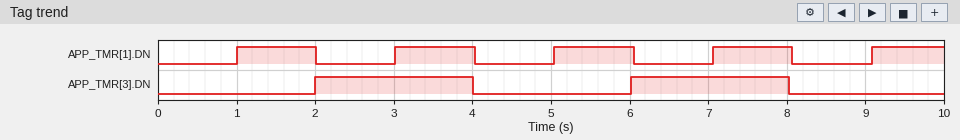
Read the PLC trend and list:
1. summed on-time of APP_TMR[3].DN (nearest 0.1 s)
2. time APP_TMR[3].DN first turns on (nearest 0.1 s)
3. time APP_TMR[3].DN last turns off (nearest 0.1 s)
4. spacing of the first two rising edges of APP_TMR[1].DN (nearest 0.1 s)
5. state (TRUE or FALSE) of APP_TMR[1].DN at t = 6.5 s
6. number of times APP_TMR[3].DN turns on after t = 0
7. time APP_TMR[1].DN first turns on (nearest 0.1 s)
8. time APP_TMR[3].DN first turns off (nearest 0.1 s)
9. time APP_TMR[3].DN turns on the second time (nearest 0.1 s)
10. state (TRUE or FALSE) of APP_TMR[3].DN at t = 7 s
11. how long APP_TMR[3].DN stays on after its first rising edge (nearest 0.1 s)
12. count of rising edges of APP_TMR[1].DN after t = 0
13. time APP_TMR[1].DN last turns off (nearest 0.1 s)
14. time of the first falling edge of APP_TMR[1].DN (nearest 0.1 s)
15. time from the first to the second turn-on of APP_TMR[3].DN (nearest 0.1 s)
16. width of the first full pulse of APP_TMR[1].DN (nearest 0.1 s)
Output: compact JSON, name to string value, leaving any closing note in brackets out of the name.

{"summed on-time of APP_TMR[3].DN": "4.0 s", "time APP_TMR[3].DN first turns on": "2.0 s", "time APP_TMR[3].DN last turns off": "8.0 s", "spacing of the first two rising edges of APP_TMR[1].DN": "2.0 s", "state (TRUE or FALSE) of APP_TMR[1].DN at t = 6.5 s": "FALSE", "number of times APP_TMR[3].DN turns on after t = 0": "2", "time APP_TMR[1].DN first turns on": "1.0 s", "time APP_TMR[3].DN first turns off": "4.0 s", "time APP_TMR[3].DN turns on the second time": "6.0 s", "state (TRUE or FALSE) of APP_TMR[3].DN at t = 7 s": "TRUE", "how long APP_TMR[3].DN stays on after its first rising edge": "2.0 s", "count of rising edges of APP_TMR[1].DN after t = 0": "5", "time APP_TMR[1].DN last turns off": "8.1 s", "time of the first falling edge of APP_TMR[1].DN": "2.0 s", "time from the first to the second turn-on of APP_TMR[3].DN": "4.0 s", "width of the first full pulse of APP_TMR[1].DN": "1.0 s"}
